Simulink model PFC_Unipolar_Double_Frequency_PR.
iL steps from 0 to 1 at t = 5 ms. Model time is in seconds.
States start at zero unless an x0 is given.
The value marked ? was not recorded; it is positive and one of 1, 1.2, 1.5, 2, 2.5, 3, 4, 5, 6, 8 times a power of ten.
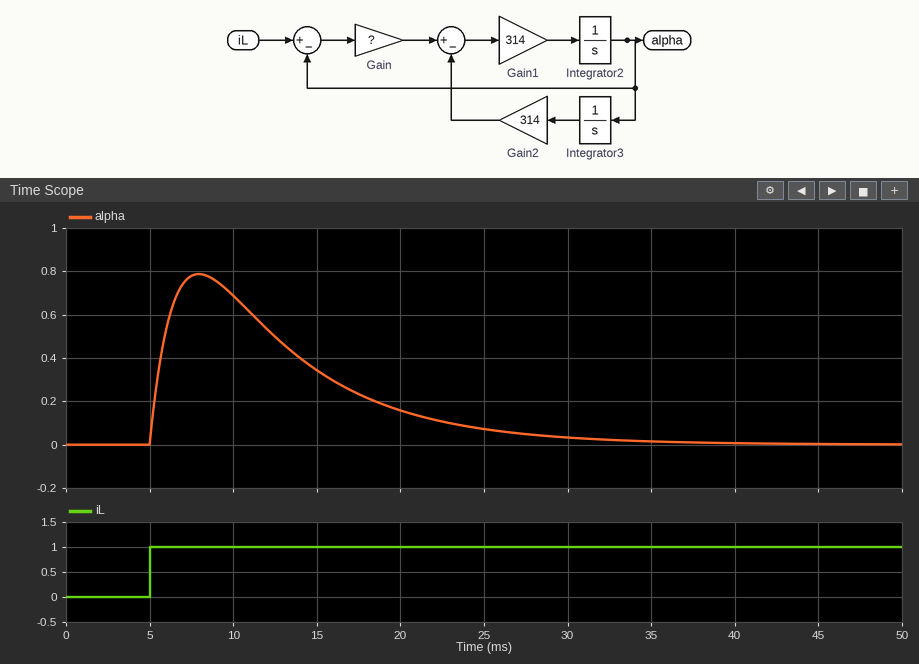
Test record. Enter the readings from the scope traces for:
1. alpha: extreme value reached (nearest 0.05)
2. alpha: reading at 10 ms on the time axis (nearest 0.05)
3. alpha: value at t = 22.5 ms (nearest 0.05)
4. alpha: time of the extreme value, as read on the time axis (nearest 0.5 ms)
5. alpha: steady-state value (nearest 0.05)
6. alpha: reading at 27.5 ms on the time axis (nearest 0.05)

0.80
0.70
0.10
8.0 ms
0.00
0.05
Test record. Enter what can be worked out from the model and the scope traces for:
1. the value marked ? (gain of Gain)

2.5
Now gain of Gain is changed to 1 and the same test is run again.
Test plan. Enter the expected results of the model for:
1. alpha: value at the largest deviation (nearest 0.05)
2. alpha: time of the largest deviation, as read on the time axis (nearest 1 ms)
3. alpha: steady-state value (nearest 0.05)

0.55
9 ms
0.00
